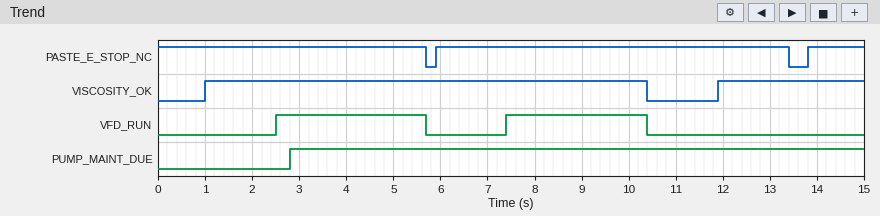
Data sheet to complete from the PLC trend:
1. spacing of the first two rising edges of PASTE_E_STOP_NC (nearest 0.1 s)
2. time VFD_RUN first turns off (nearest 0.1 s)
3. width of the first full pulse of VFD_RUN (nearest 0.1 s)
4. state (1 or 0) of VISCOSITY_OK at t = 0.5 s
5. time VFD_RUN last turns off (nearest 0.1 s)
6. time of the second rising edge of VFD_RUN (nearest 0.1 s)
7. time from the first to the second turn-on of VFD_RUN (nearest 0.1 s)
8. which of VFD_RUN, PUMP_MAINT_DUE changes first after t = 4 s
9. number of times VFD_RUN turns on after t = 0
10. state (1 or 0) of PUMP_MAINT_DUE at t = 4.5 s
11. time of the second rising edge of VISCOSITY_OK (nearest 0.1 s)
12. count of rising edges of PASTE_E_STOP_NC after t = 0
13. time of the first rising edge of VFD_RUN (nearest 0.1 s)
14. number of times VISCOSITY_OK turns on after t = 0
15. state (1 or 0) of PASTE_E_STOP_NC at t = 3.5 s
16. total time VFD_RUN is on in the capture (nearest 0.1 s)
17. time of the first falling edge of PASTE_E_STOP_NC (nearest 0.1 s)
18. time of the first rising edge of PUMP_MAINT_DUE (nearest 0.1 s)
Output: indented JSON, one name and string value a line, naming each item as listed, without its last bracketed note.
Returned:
{
  "spacing of the first two rising edges of PASTE_E_STOP_NC": "7.9 s",
  "time VFD_RUN first turns off": "5.7 s",
  "width of the first full pulse of VFD_RUN": "3.2 s",
  "state (1 or 0) of VISCOSITY_OK at t = 0.5 s": "0",
  "time VFD_RUN last turns off": "10.4 s",
  "time of the second rising edge of VFD_RUN": "7.4 s",
  "time from the first to the second turn-on of VFD_RUN": "4.9 s",
  "which of VFD_RUN, PUMP_MAINT_DUE changes first after t = 4 s": "VFD_RUN",
  "number of times VFD_RUN turns on after t = 0": "2",
  "state (1 or 0) of PUMP_MAINT_DUE at t = 4.5 s": "1",
  "time of the second rising edge of VISCOSITY_OK": "11.9 s",
  "count of rising edges of PASTE_E_STOP_NC after t = 0": "2",
  "time of the first rising edge of VFD_RUN": "2.5 s",
  "number of times VISCOSITY_OK turns on after t = 0": "2",
  "state (1 or 0) of PASTE_E_STOP_NC at t = 3.5 s": "1",
  "total time VFD_RUN is on in the capture": "6.2 s",
  "time of the first falling edge of PASTE_E_STOP_NC": "5.7 s",
  "time of the first rising edge of PUMP_MAINT_DUE": "2.8 s"
}
